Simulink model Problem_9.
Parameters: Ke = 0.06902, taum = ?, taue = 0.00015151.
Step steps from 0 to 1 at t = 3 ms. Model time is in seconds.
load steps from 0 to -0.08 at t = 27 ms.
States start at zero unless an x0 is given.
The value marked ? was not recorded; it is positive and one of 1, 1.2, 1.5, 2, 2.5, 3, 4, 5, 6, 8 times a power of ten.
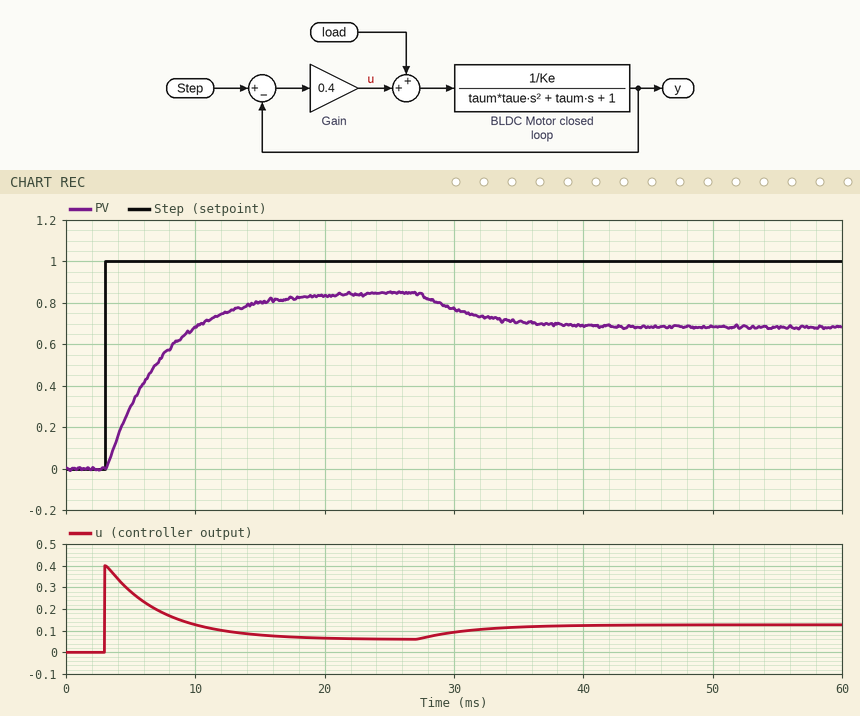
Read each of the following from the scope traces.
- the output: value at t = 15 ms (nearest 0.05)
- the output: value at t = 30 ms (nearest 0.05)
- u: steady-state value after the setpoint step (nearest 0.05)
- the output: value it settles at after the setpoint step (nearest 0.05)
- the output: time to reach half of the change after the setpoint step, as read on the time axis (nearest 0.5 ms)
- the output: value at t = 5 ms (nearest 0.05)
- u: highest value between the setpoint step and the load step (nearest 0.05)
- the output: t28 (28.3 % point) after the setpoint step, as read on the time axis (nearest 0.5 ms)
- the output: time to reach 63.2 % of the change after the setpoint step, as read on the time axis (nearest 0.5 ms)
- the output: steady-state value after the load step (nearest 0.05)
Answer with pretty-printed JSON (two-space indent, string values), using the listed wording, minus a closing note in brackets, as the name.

{
  "the output: value at t = 15 ms": "0.80",
  "the output: value at t = 30 ms": "0.75",
  "u: steady-state value after the setpoint step": "0.05",
  "the output: value it settles at after the setpoint step": "0.85",
  "the output: time to reach half of the change after the setpoint step, as read on the time axis": "6.0 ms",
  "the output: value at t = 5 ms": "0.30",
  "u: highest value between the setpoint step and the load step": "0.40",
  "the output: t28 (28.3 % point) after the setpoint step, as read on the time axis": "4.5 ms",
  "the output: time to reach 63.2 % of the change after the setpoint step, as read on the time axis": "7.5 ms",
  "the output: steady-state value after the load step": "0.70"
}
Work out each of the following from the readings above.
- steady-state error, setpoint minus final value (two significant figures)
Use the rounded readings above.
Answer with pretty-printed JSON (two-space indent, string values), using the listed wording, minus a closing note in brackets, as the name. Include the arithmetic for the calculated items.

{
  "steady-state error, setpoint minus final value": "1 - 0.85 = 0.15"
}
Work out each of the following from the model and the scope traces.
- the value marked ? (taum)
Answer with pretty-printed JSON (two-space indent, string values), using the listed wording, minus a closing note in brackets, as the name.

{
  "the value marked ?": "0.03"
}
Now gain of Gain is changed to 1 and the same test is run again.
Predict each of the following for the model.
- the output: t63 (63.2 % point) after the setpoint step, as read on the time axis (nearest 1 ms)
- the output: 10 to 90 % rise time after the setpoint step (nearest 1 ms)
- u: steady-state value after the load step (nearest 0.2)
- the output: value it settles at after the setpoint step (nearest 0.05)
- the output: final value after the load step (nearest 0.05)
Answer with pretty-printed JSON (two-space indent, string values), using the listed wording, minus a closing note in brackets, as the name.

{
  "the output: t63 (63.2 % point) after the setpoint step, as read on the time axis": "5 ms",
  "the output: 10 to 90 % rise time after the setpoint step": "4 ms",
  "u: steady-state value after the load step": "0.2",
  "the output: value it settles at after the setpoint step": "0.95",
  "the output: final value after the load step": "0.85"
}
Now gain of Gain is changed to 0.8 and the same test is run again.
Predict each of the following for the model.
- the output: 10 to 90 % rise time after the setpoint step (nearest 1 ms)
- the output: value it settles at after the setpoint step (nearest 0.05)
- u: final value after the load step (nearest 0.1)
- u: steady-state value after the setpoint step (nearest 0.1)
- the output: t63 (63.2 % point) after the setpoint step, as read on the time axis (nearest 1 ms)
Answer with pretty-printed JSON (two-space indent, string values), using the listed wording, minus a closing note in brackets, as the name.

{
  "the output: 10 to 90 % rise time after the setpoint step": "5 ms",
  "the output: value it settles at after the setpoint step": "0.90",
  "u: final value after the load step": "0.1",
  "u: steady-state value after the setpoint step": "0.1",
  "the output: t63 (63.2 % point) after the setpoint step, as read on the time axis": "5 ms"
}
